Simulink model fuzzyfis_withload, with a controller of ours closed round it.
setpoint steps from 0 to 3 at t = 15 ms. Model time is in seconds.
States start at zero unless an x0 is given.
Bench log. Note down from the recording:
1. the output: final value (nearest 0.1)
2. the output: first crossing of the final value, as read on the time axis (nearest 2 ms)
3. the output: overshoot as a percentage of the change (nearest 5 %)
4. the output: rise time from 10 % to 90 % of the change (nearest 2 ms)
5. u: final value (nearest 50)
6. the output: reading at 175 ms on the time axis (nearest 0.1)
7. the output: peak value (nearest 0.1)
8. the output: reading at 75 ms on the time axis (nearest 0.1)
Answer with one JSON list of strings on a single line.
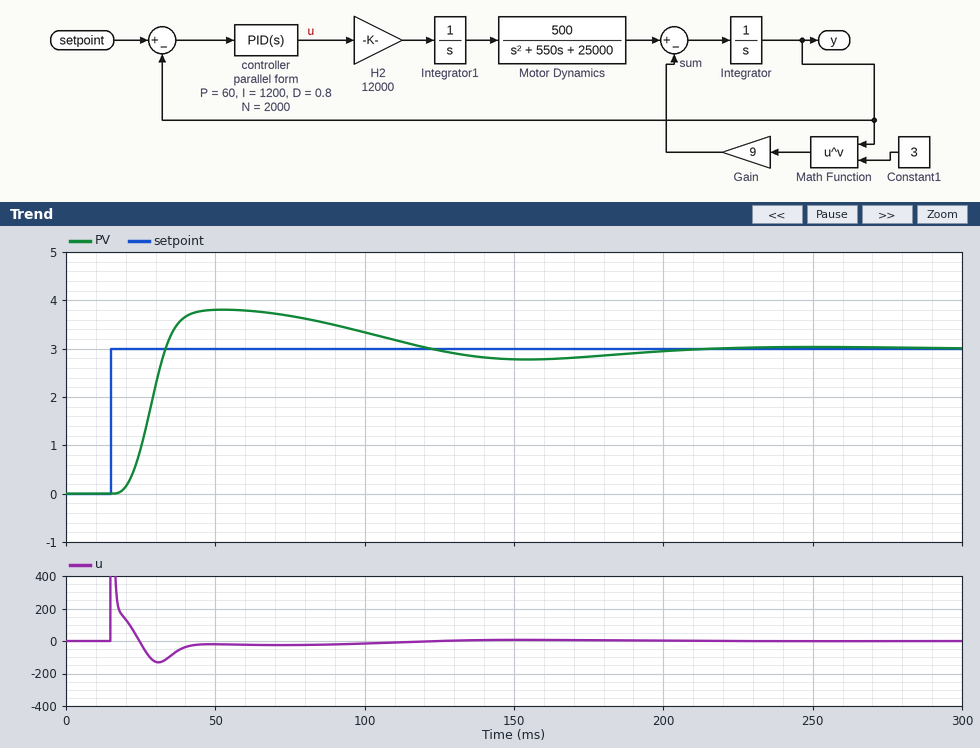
["3.0", "34 ms", "25 %", "10 ms", "0", "2.8", "3.8", "3.7"]
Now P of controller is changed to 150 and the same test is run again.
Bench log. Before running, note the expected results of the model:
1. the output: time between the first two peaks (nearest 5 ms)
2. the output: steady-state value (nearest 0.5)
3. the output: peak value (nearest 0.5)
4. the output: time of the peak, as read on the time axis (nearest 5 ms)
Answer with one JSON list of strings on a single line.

["80 ms", "3.0", "4.5", "45 ms"]
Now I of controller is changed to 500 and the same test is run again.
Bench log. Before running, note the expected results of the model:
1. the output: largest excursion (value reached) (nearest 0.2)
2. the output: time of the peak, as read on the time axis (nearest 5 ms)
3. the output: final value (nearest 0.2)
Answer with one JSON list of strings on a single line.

["3.6", "45 ms", "3.0"]
